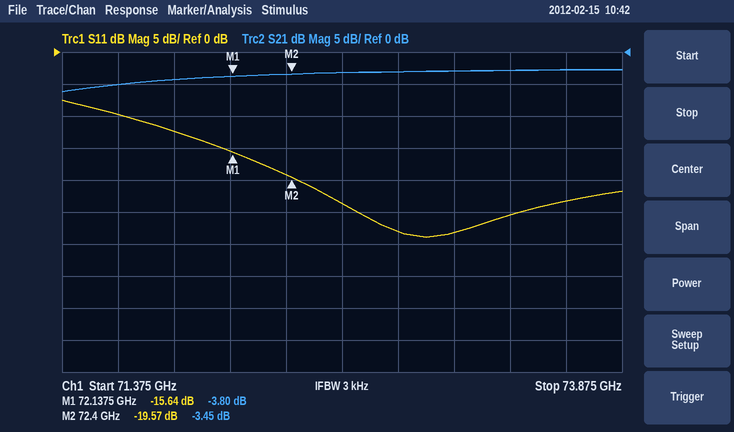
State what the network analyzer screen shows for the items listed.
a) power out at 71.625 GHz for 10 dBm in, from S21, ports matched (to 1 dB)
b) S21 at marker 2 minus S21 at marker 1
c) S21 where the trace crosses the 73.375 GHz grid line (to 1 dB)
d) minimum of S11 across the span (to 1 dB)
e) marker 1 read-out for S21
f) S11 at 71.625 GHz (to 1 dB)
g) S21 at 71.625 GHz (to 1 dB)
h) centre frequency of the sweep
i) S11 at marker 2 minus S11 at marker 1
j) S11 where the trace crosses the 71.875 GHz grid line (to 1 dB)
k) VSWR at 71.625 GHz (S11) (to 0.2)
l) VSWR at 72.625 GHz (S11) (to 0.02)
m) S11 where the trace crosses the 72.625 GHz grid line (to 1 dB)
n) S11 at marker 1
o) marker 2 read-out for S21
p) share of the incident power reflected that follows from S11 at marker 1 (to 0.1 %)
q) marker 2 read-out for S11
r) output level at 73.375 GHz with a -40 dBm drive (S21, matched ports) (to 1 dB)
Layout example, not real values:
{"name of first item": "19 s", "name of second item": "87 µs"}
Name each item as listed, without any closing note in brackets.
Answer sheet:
{"power out at 71.625 GHz for 10 dBm in, from S21, ports matched": "5 dBm", "S21 at marker 2 minus S21 at marker 1": "0.35 dB", "S21 where the trace crosses the 73.375 GHz grid line": "-3 dB", "minimum of S11 across the span": "-29 dB", "marker 1 read-out for S21": "-3.80 dB", "S11 at 71.625 GHz": "-10 dB", "S21 at 71.625 GHz": "-5 dB", "centre frequency of the sweep": "72.625 GHz", "S11 at marker 2 minus S11 at marker 1": "-3.93 dB", "S11 where the trace crosses the 71.875 GHz grid line": "-12 dB", "VSWR at 71.625 GHz (S11)": "2.0", "VSWR at 72.625 GHz (S11)": "1.14", "S11 where the trace crosses the 72.625 GHz grid line": "-24 dB", "S11 at marker 1": "-15.64 dB", "marker 2 read-out for S21": "-3.45 dB", "share of the incident power reflected that follows from S11 at marker 1": "2.7 %", "marker 2 read-out for S11": "-19.57 dB", "output level at 73.375 GHz with a -40 dBm drive (S21, matched ports)": "-43 dBm"}
